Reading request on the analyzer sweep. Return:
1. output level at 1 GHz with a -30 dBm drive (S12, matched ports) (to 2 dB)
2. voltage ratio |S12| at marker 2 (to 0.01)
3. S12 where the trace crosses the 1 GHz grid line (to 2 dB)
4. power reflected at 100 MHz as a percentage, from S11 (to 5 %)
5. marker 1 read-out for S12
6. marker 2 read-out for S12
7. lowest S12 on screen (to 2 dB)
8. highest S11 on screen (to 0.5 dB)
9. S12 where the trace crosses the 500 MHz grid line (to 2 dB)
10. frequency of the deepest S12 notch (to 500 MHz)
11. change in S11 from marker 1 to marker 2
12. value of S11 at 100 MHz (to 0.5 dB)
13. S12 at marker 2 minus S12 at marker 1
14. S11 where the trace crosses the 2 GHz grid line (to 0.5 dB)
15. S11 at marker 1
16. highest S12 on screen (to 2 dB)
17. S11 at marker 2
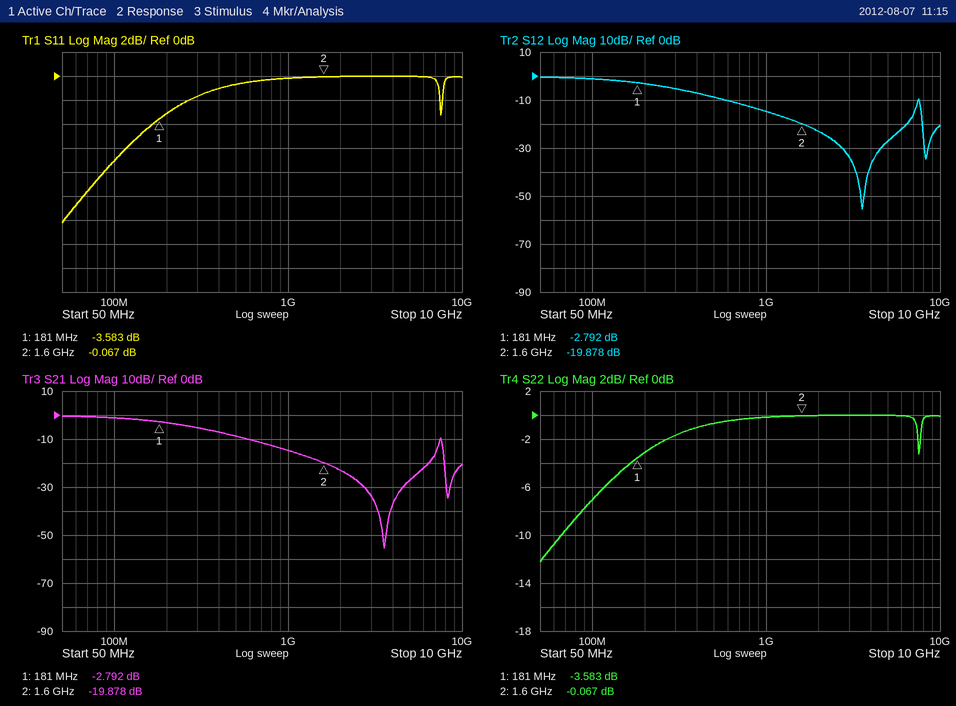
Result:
-44 dBm
0.10
-14 dB
20 %
-2.792 dB
-19.878 dB
-56 dB
0.0 dB
-8 dB
3.5 GHz
3.516 dB
-7.0 dB
-17.086 dB
0.0 dB
-3.583 dB
0 dB
-0.067 dB
